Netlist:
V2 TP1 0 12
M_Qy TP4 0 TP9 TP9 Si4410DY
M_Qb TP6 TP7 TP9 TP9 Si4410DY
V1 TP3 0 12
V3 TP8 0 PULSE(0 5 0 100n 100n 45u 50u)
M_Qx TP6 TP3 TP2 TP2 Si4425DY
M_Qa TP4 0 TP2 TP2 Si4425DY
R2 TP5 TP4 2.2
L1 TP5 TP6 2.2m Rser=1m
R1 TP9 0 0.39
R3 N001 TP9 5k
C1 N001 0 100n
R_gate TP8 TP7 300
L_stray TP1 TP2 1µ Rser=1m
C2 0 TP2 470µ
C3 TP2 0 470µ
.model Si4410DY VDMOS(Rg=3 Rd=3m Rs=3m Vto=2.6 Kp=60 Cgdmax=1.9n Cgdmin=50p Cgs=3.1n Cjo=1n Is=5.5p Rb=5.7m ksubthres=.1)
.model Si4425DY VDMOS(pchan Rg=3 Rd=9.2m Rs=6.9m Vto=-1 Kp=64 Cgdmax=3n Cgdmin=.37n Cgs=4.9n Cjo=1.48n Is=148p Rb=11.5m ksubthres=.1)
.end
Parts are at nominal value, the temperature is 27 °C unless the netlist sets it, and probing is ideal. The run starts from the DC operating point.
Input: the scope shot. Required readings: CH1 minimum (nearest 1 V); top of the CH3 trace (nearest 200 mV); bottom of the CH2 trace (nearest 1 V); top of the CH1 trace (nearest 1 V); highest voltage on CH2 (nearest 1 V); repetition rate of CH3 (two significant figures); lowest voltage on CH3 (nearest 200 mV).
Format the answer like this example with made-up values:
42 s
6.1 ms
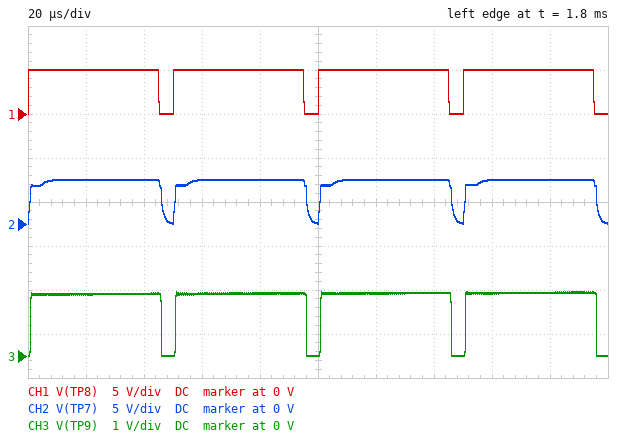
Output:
0 V
1.4 V
0 V
5 V
5 V
20 kHz
0 V
